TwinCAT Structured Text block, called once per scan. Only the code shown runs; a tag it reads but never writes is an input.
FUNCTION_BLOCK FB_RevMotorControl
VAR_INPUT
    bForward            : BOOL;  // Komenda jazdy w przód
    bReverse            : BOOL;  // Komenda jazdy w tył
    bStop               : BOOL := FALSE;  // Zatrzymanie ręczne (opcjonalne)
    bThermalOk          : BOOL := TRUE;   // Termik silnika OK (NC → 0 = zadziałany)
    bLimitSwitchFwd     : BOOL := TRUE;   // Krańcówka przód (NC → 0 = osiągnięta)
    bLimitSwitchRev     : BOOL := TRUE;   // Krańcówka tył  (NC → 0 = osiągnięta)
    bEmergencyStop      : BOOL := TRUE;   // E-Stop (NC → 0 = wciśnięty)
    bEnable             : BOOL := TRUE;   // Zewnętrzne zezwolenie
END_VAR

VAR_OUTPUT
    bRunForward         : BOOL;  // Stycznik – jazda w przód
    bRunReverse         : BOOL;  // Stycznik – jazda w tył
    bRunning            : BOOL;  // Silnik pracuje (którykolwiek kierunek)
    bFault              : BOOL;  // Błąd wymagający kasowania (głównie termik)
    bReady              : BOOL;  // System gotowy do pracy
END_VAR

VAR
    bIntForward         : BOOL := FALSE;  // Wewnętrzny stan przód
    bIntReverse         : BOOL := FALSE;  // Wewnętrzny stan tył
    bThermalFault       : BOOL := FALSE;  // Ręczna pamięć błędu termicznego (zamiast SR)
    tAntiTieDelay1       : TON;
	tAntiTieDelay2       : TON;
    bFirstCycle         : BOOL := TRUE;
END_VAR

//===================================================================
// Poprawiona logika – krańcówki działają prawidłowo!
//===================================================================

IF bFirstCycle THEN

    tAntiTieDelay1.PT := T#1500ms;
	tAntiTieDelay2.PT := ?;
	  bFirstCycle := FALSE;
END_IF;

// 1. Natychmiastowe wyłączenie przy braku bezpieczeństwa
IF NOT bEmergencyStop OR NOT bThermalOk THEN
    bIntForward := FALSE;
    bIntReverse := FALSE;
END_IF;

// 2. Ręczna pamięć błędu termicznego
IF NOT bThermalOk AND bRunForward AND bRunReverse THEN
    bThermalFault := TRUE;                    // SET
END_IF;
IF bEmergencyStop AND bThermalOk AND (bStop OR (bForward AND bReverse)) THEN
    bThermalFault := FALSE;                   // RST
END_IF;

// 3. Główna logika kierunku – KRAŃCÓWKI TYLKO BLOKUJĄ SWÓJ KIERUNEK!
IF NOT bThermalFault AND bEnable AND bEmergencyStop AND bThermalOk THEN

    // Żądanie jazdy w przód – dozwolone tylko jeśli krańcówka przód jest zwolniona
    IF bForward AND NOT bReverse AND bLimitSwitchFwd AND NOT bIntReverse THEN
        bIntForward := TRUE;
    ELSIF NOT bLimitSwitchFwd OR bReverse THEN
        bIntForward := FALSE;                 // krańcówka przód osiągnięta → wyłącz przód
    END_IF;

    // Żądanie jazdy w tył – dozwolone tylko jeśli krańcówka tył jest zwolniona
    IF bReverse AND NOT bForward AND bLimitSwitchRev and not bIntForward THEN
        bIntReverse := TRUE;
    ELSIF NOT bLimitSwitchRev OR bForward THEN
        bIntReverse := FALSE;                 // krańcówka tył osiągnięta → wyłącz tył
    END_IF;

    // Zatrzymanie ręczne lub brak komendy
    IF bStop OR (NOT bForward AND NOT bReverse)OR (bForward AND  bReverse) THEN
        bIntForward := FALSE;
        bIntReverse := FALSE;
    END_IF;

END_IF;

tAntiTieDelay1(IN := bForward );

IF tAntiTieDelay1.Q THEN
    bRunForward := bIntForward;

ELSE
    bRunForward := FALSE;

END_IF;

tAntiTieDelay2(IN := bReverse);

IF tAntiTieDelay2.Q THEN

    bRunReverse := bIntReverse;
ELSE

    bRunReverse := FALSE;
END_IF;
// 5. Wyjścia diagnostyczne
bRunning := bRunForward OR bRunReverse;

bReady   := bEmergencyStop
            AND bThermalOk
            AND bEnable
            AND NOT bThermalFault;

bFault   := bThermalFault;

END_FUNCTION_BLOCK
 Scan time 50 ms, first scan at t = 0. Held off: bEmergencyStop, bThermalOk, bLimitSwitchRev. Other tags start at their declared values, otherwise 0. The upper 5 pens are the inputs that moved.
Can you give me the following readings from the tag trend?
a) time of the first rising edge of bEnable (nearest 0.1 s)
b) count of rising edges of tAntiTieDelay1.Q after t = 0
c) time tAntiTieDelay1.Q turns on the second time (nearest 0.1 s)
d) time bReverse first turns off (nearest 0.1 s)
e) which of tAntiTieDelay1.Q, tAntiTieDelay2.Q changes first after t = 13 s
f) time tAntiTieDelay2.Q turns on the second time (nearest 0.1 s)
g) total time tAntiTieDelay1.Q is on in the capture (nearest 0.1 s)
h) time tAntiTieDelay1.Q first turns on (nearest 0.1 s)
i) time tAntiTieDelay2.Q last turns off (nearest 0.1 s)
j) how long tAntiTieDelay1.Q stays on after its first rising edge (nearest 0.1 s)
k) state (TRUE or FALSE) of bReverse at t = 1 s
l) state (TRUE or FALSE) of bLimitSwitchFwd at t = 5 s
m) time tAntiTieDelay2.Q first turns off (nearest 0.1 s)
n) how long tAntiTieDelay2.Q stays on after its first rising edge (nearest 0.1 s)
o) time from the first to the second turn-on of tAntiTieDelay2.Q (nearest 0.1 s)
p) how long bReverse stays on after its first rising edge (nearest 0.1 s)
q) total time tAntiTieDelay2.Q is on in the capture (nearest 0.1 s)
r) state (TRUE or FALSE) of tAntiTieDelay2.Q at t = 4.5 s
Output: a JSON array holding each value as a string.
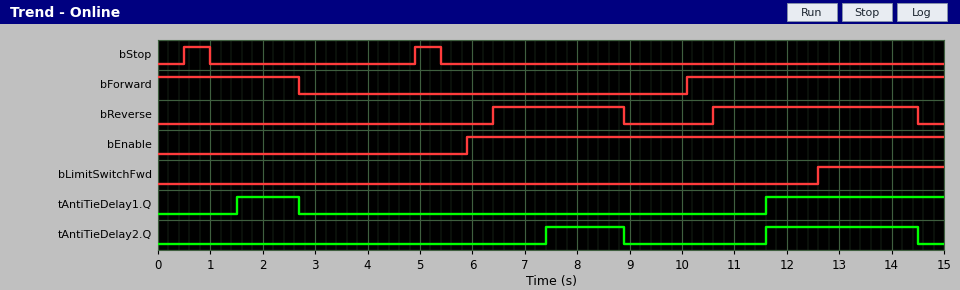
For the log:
["5.9 s", "2", "11.6 s", "8.9 s", "tAntiTieDelay2.Q", "11.6 s", "4.6 s", "1.5 s", "14.5 s", "1.2 s", "FALSE", "FALSE", "8.9 s", "1.5 s", "4.2 s", "2.5 s", "4.4 s", "FALSE"]
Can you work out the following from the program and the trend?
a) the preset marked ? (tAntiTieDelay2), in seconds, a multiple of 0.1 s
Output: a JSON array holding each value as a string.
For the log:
["1.0 s"]
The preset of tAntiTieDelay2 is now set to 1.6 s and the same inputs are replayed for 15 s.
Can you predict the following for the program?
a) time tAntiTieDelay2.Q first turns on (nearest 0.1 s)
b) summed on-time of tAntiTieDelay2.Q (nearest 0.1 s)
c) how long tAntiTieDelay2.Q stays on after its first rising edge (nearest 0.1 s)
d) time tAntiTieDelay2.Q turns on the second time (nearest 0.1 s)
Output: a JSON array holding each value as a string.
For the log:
["8.0 s", "3.2 s", "0.9 s", "12.2 s"]
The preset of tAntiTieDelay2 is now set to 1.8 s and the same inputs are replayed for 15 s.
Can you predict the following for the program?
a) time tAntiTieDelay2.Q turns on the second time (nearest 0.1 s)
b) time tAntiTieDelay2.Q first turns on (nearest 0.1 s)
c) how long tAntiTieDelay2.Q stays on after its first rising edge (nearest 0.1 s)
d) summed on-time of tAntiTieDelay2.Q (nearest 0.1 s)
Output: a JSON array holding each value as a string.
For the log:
["12.4 s", "8.2 s", "0.7 s", "2.8 s"]
